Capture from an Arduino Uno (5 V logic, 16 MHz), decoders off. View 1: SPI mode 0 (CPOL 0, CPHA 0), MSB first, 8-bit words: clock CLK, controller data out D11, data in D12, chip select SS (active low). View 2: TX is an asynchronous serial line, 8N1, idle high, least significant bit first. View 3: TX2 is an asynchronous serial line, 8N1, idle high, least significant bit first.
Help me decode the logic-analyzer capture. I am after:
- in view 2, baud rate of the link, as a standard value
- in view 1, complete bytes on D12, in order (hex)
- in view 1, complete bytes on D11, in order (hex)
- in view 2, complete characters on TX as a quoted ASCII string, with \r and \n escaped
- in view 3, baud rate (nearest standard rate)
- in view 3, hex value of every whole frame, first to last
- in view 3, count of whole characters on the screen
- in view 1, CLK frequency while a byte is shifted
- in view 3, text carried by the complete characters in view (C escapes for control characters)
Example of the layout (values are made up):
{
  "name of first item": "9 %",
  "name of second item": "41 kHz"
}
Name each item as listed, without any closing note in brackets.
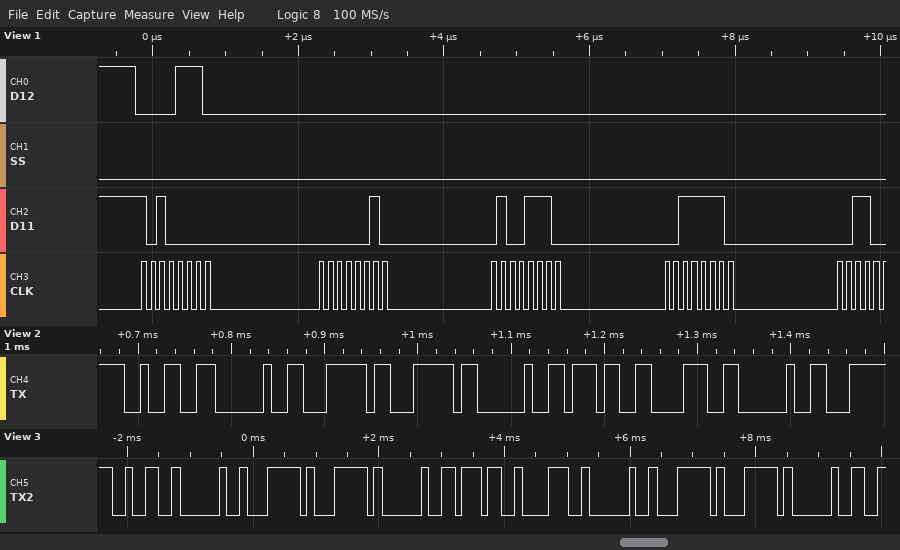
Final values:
{
  "in view 2, baud rate of the link, as a standard value": "115200 baud",
  "in view 1, complete bytes on D12, in order": "0E 00 00 00",
  "in view 1, complete bytes on D11, in order": "A0 02 4E 3E",
  "in view 2, complete characters on TX as a quoted ASCII string, with \\r and \\n escaped": "\"2 || 78 \"",
  "in view 3, baud rate": "9600 baud",
  "in view 3, hex value of every whole frame, first to last": "32 20 7C 7C 20 37 38 20 7C 7C 20",
  "in view 3, count of whole characters on the screen": "11",
  "in view 1, CLK frequency while a byte is shifted": "8 MHz",
  "in view 3, text carried by the complete characters in view": "\"2 || 78 || \""
}
